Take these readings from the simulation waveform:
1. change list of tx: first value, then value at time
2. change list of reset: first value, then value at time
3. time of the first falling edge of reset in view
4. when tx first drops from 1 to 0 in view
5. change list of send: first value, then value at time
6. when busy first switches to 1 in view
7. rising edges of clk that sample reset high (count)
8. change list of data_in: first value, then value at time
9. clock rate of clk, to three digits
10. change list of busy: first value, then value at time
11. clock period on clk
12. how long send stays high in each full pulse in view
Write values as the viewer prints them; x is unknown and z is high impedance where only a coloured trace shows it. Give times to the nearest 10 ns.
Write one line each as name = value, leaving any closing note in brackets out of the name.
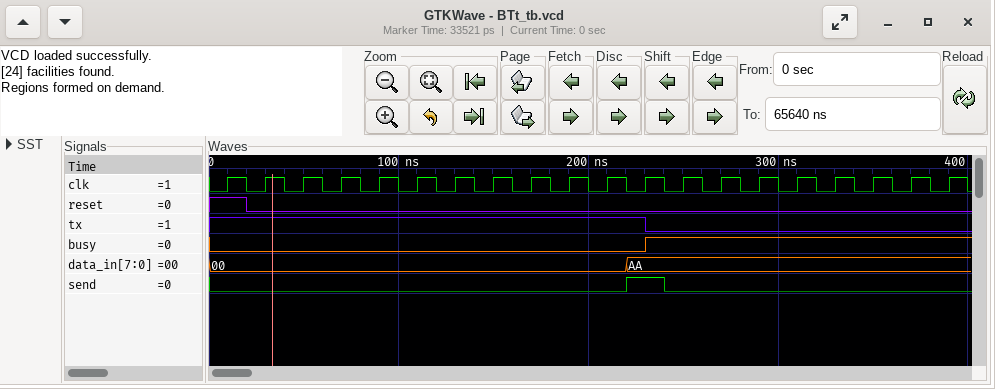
change list of tx: first value, then value at time = 1, 0 at 230 ns
change list of reset: first value, then value at time = 1, 0 at 20 ns
time of the first falling edge of reset in view = 20 ns
when tx first drops from 1 to 0 in view = 230 ns
change list of send: first value, then value at time = 0, 1 at 220 ns, 0 at 240 ns
when busy first switches to 1 in view = 230 ns
rising edges of clk that sample reset high = 1
change list of data_in: first value, then value at time = 00, AA at 220 ns
clock rate of clk, to three digits = 50.0 MHz
change list of busy: first value, then value at time = 0, 1 at 230 ns
clock period on clk = 20 ns
how long send stays high in each full pulse in view = 20 ns
